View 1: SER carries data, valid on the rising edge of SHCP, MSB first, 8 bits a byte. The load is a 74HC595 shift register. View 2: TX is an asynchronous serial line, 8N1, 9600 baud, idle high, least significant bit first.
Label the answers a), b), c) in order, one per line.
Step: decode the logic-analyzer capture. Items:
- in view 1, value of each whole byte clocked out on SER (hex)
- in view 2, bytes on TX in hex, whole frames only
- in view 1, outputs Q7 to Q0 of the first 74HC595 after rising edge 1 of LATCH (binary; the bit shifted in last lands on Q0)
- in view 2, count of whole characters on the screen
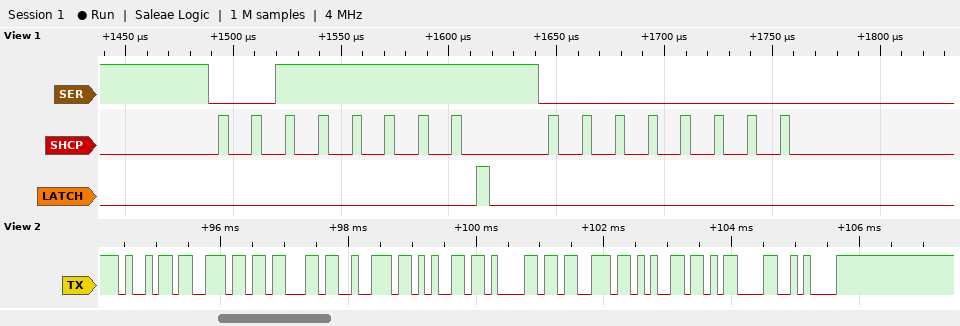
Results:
a) 0x3F 0x00
b) 69 6E 63 72 65 61 73 65 0D 0A
c) 00111111
d) 10
